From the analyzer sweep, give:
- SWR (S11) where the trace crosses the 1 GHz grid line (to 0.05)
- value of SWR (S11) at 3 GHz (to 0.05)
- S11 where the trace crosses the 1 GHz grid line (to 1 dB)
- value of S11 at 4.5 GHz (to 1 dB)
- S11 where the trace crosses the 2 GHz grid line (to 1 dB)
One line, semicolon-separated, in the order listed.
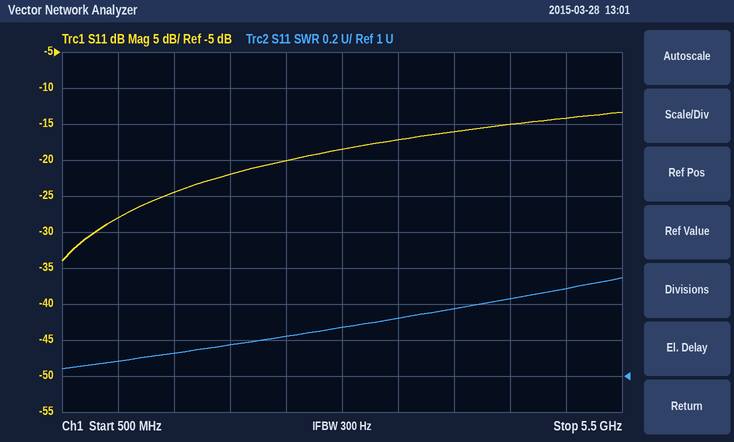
1.10; 1.25; -28 dB; -15 dB; -22 dB
